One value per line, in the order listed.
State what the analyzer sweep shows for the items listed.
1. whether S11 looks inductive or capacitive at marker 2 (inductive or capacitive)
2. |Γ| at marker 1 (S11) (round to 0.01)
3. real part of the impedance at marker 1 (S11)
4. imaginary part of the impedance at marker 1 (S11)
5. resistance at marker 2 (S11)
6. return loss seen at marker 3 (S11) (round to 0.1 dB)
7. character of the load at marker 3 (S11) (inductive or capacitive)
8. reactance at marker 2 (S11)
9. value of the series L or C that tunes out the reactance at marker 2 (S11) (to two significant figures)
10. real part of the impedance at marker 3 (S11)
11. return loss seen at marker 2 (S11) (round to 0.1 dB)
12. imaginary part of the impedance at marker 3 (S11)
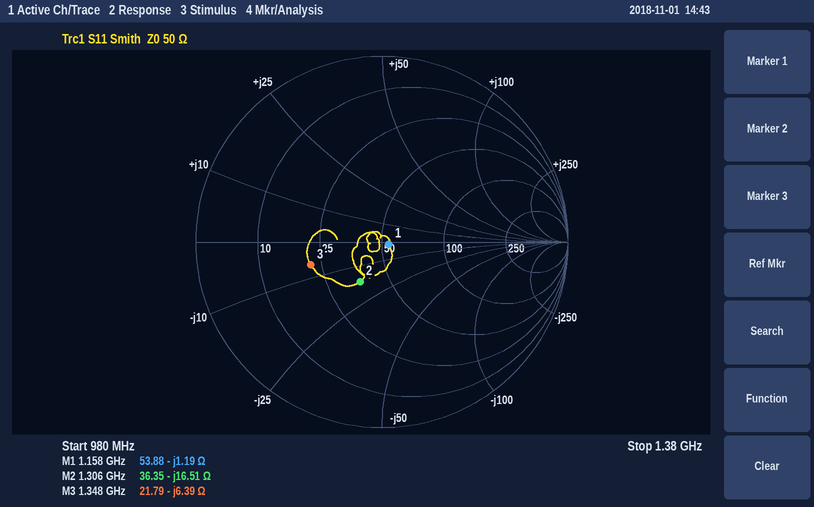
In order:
capacitive
0.04
53.88 Ω
-1.19 Ω
36.35 Ω
7.9 dB
capacitive
-16.51 Ω
2.0 nH
21.79 Ω
12.3 dB
-6.39 Ω
